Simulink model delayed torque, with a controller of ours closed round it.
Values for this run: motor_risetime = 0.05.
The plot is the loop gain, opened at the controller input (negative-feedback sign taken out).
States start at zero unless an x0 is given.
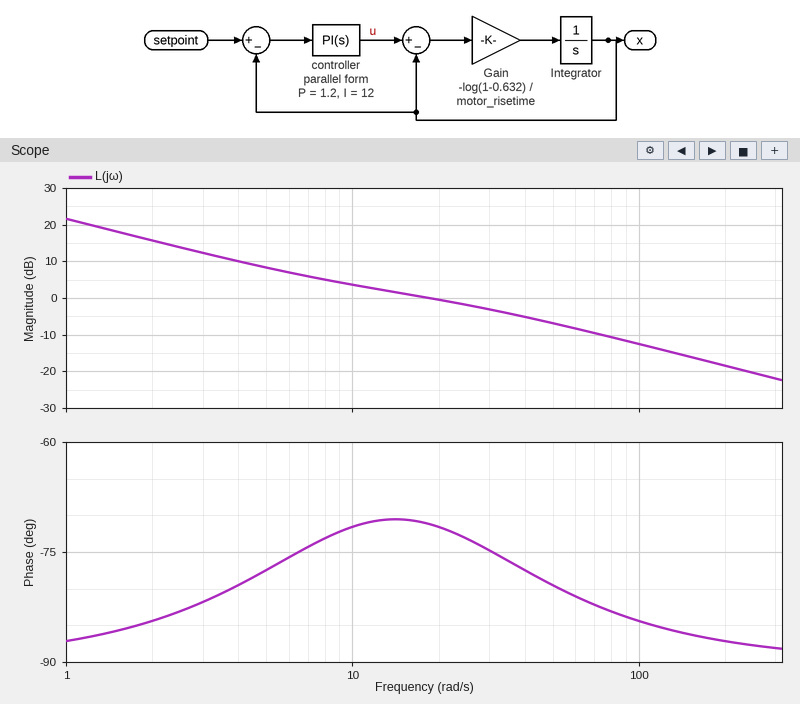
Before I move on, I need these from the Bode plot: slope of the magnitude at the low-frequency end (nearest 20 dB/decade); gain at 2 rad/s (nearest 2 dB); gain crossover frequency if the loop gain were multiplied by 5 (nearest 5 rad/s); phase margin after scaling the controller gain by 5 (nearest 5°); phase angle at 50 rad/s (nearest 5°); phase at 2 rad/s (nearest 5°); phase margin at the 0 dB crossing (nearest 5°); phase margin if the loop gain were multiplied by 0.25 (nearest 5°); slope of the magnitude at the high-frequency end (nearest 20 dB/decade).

-20 dB/decade
16 dB
120 rad/s
95°
-80°
-85°
110°
100°
-20 dB/decade
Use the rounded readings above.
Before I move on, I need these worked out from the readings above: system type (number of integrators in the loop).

1
